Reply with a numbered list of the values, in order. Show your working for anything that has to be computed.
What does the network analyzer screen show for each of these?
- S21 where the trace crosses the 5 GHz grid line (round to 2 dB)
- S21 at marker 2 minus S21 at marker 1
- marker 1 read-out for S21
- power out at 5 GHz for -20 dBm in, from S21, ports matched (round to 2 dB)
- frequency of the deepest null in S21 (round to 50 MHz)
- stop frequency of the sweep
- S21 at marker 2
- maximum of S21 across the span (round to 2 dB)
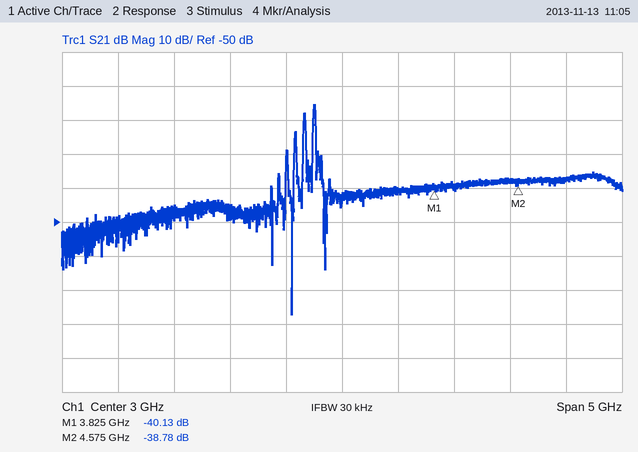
1. -38 dB
2. -38.78 − (-40.13) = 1.35 dB
3. -40.13 dB
4. -20 dBm + (-38 dB) = -58 dBm
5. 2.55 GHz
6. 5.5 GHz
7. -38.78 dB
8. -16 dB
